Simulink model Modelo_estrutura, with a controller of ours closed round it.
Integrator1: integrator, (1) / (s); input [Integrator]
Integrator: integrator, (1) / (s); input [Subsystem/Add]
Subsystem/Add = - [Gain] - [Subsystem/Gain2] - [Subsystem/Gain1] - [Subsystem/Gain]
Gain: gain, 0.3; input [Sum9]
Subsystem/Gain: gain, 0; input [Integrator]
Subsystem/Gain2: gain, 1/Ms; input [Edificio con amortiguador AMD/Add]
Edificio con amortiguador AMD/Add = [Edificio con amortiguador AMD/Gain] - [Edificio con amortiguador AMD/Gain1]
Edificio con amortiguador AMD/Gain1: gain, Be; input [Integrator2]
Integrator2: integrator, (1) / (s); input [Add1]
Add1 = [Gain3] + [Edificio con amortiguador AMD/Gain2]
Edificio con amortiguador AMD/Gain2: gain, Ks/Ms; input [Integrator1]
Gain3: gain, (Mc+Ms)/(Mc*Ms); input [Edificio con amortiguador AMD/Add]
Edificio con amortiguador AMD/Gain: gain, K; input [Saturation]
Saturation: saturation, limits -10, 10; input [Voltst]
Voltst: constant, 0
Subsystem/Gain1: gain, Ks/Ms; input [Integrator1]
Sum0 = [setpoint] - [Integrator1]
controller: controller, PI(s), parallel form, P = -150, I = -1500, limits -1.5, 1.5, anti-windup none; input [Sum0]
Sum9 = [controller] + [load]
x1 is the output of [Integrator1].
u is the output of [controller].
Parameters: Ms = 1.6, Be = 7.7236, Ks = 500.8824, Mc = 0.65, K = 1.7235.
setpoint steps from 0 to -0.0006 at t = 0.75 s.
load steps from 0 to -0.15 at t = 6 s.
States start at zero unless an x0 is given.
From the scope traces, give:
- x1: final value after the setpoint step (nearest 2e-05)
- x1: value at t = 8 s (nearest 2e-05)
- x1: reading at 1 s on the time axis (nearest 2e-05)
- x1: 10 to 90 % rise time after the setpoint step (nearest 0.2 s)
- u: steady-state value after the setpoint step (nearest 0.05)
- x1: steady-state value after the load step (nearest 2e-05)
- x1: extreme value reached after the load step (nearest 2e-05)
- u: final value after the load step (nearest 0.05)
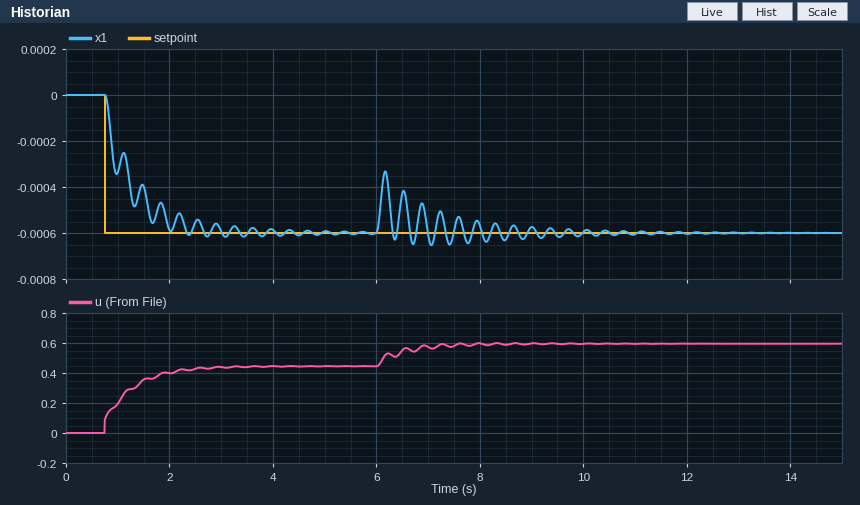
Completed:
-0.00060
-0.00056
-0.00034
0.8 s
0.45
-0.00060
-0.00034
0.60
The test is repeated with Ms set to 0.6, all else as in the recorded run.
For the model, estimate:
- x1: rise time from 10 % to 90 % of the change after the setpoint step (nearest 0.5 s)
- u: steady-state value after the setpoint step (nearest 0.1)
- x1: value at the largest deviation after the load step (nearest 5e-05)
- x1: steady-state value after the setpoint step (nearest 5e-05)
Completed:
2.0 s
0.8
-0.00045
-0.00060
